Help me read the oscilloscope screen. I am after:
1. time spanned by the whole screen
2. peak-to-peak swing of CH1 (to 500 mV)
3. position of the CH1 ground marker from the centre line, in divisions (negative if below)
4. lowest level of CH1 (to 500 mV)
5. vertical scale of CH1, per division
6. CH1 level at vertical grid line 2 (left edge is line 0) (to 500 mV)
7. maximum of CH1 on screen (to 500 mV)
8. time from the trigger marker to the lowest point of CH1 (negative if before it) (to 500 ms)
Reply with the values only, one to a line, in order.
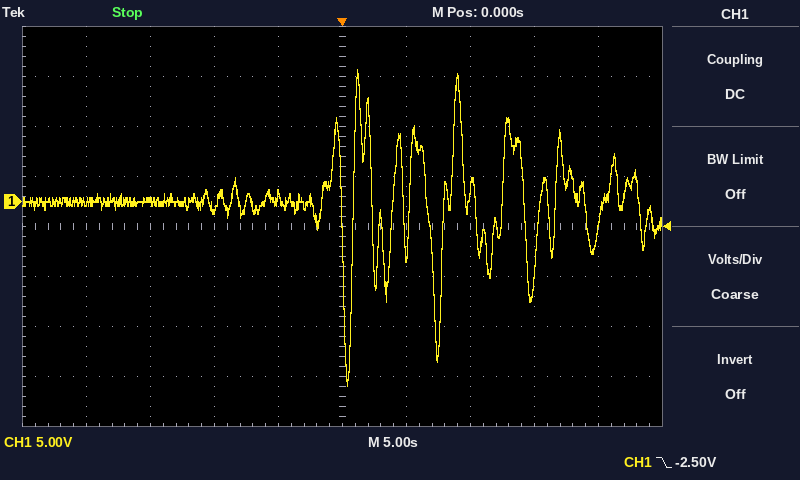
50 s
31.5 V
+0.5 div
-18.5 V
5 V
0.0 V
13.0 V
+500 ms
